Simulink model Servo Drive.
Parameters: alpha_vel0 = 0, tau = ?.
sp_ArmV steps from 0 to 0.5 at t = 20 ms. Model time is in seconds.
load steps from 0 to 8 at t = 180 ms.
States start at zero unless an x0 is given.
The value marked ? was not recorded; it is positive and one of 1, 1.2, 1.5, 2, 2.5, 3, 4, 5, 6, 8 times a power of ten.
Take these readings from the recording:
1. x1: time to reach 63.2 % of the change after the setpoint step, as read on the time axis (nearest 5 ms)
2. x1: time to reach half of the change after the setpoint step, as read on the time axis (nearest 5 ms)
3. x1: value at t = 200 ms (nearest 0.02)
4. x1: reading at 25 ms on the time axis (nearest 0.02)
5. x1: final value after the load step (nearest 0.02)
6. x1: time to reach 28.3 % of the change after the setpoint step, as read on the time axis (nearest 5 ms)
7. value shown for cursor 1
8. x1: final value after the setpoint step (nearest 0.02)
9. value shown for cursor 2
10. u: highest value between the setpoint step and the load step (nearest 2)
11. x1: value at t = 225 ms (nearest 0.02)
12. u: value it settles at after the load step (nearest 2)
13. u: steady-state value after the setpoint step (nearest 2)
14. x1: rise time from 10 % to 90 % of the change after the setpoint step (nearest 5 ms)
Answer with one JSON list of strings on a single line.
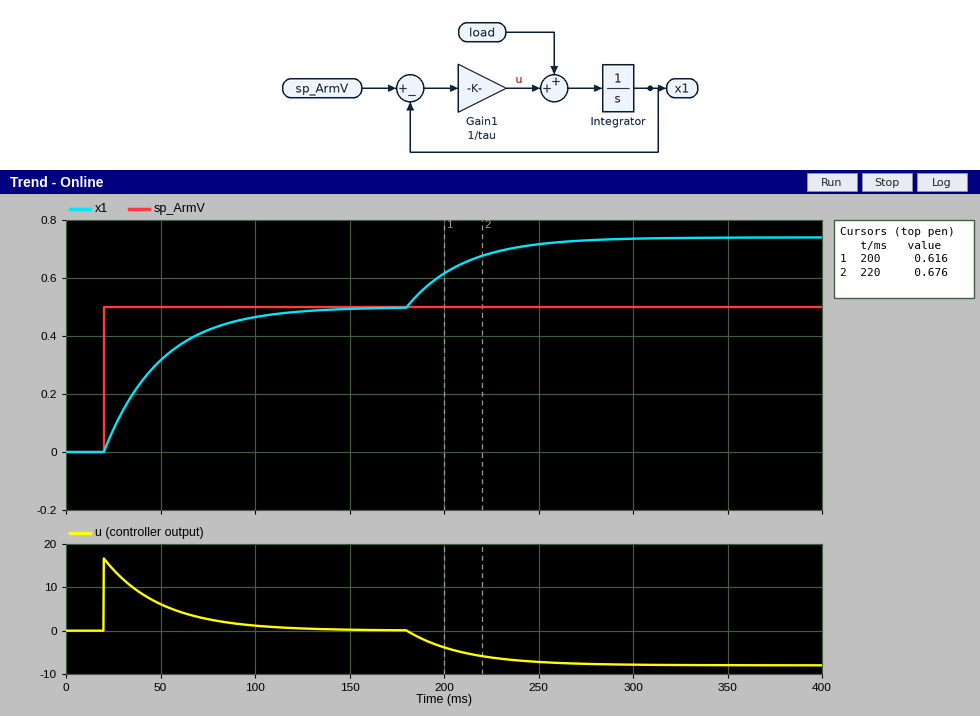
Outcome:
["50 ms", "40 ms", "0.62", "0.08", "0.74", "30 ms", "0.616", "0.50", "0.676", "16", "0.68", "-8", "0", "65 ms"]
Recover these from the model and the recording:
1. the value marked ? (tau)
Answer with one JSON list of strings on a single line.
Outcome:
["0.03"]
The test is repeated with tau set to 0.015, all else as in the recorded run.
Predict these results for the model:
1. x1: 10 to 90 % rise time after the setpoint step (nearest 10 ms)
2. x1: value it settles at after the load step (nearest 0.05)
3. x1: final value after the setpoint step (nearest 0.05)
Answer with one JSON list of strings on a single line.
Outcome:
["30 ms", "0.60", "0.50"]
